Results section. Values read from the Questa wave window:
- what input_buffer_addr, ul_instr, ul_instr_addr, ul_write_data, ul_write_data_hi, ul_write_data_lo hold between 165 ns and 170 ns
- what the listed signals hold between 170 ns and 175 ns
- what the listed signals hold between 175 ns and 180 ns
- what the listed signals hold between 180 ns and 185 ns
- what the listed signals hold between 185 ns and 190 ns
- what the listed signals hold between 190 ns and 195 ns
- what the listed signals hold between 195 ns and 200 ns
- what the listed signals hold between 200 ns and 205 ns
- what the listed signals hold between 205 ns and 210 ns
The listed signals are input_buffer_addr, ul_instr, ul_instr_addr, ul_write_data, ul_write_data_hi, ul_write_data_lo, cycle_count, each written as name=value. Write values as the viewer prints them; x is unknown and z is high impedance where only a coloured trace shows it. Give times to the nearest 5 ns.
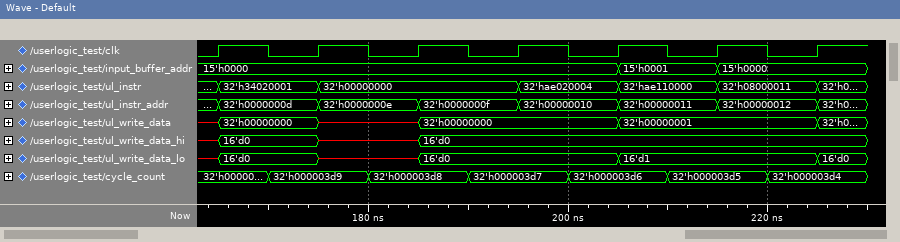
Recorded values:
input_buffer_addr=15'h0000, ul_instr=32'h34020001, ul_instr_addr=32'h0000000d, ul_write_data=32'h00000000, ul_write_data_hi=16'd0, ul_write_data_lo=16'd0
input_buffer_addr=15'h0000, ul_instr=32'h34020001, ul_instr_addr=32'h0000000d, ul_write_data=32'h00000000, ul_write_data_hi=16'd0, ul_write_data_lo=16'd0, cycle_count=32'h000003d9
input_buffer_addr=15'h0000, ul_instr=32'h00000000, ul_instr_addr=32'h0000000e, ul_write_data=x, ul_write_data_hi=x, ul_write_data_lo=x, cycle_count=32'h000003d9
input_buffer_addr=15'h0000, ul_instr=32'h00000000, ul_instr_addr=32'h0000000e, ul_write_data=x, ul_write_data_hi=x, ul_write_data_lo=x, cycle_count=32'h000003d8
input_buffer_addr=15'h0000, ul_instr=32'h00000000, ul_instr_addr=32'h0000000f, ul_write_data=32'h00000000, ul_write_data_hi=16'd0, ul_write_data_lo=16'd0, cycle_count=32'h000003d8
input_buffer_addr=15'h0000, ul_instr=32'h00000000, ul_instr_addr=32'h0000000f, ul_write_data=32'h00000000, ul_write_data_hi=16'd0, ul_write_data_lo=16'd0, cycle_count=32'h000003d7
input_buffer_addr=15'h0000, ul_instr=32'hae020004, ul_instr_addr=32'h00000010, ul_write_data=32'h00000000, ul_write_data_hi=16'd0, ul_write_data_lo=16'd0, cycle_count=32'h000003d7
input_buffer_addr=15'h0000, ul_instr=32'hae020004, ul_instr_addr=32'h00000010, ul_write_data=32'h00000000, ul_write_data_hi=16'd0, ul_write_data_lo=16'd0, cycle_count=32'h000003d6
input_buffer_addr=15'h0001, ul_instr=32'hae110000, ul_instr_addr=32'h00000011, ul_write_data=32'h00000001, ul_write_data_hi=16'd0, ul_write_data_lo=16'd1, cycle_count=32'h000003d6
